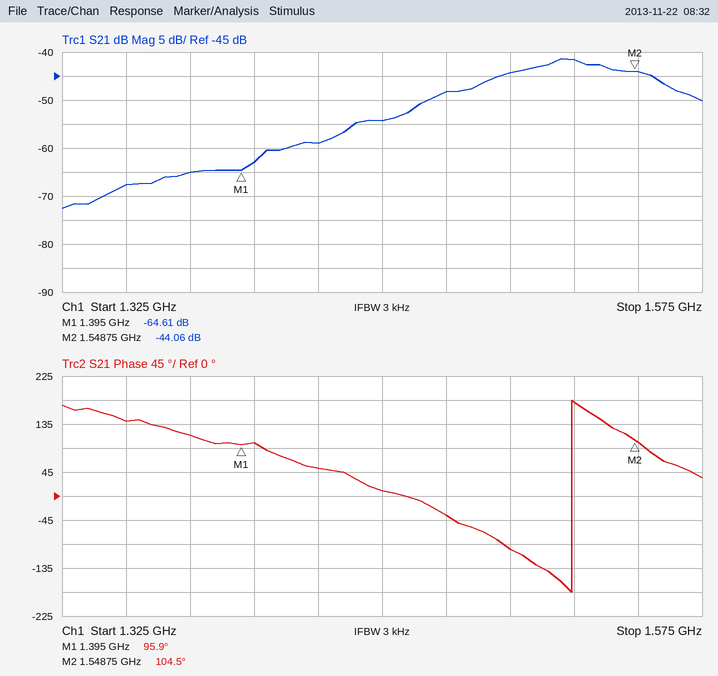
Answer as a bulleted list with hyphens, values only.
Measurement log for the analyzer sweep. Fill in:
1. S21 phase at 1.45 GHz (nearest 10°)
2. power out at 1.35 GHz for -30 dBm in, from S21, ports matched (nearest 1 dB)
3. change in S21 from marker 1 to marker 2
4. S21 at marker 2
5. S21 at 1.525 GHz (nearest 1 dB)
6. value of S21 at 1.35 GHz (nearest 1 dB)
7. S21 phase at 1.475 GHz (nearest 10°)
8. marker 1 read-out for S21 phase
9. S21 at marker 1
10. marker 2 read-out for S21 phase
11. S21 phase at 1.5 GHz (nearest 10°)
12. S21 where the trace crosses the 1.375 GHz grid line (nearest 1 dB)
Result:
- 10°
- -98 dBm
- 20.55 dB
- -44.06 dB
- -42 dB
- -68 dB
- -40°
- 95.9°
- -64.61 dB
- 104.5°
- -100°
- -65 dB
